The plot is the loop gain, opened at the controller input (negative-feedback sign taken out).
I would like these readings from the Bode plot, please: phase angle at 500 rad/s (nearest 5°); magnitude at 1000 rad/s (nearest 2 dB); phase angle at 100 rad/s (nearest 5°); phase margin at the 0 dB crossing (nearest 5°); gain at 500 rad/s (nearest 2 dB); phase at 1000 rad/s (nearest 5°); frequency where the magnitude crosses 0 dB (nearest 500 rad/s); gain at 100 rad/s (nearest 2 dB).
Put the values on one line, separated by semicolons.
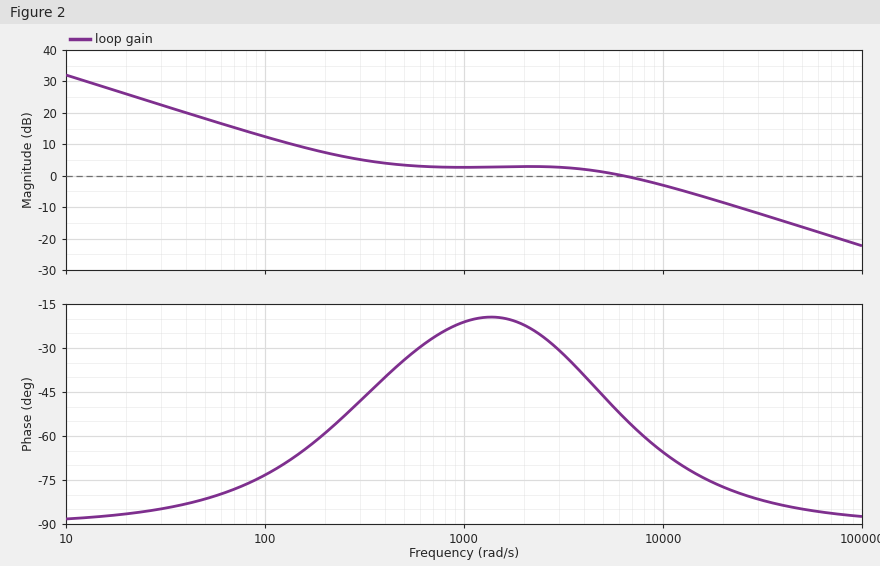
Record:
-35°; 2 dB; -75°; 125°; 4 dB; -20°; 6500 rad/s; 12 dB
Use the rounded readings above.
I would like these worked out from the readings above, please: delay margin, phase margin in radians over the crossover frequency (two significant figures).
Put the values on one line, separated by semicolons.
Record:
0.00034 s
